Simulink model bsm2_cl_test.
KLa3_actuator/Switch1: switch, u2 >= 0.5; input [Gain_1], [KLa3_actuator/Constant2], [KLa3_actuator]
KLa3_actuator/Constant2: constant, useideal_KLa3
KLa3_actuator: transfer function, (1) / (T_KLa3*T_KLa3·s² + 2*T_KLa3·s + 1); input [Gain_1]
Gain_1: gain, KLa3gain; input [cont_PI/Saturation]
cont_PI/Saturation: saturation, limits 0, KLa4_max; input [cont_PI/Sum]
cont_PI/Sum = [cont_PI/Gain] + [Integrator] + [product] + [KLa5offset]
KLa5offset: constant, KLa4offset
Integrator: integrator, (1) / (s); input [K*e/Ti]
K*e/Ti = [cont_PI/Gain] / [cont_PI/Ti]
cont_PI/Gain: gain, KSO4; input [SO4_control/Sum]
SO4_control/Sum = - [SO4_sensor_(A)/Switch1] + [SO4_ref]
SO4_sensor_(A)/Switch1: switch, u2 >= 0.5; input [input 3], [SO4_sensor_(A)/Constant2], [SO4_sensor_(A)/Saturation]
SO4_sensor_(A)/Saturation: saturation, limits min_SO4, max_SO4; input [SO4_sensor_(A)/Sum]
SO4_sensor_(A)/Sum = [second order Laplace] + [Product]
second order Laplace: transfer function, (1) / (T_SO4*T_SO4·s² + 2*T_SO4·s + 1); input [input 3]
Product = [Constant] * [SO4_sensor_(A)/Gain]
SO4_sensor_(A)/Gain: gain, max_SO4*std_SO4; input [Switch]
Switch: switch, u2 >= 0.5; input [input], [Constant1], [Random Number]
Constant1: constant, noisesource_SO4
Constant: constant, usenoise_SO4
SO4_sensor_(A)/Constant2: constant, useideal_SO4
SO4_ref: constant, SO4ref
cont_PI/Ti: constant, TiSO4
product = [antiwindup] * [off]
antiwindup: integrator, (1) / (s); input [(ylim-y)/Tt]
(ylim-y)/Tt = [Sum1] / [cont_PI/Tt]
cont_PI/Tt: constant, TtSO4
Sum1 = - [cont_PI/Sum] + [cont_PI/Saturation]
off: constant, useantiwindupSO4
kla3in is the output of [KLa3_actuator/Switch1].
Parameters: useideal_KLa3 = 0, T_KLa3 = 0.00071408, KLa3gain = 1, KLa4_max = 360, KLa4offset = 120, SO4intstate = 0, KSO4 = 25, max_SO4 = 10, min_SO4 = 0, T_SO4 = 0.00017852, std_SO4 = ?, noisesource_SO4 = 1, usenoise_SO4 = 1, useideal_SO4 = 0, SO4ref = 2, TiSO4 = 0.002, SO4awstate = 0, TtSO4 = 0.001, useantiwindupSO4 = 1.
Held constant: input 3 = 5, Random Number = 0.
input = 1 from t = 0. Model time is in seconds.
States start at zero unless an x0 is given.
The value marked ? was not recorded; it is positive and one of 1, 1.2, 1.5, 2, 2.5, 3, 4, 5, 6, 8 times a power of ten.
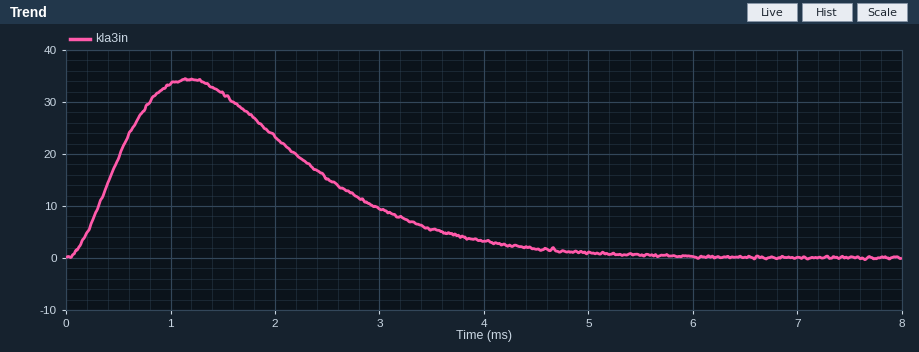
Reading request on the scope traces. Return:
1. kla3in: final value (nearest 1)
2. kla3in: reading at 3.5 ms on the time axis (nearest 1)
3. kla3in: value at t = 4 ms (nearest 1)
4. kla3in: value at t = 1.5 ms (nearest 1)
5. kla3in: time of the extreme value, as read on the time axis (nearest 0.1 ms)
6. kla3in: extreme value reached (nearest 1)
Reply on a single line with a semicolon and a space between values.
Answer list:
0; 6; 3; 32; 1.2 ms; 34
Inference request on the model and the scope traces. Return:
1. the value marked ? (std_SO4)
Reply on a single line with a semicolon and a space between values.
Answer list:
0.05
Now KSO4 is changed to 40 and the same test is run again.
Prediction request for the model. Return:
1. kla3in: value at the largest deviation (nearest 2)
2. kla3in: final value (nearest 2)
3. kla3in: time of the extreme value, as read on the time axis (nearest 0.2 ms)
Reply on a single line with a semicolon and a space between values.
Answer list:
26; 0; 1.0 ms
